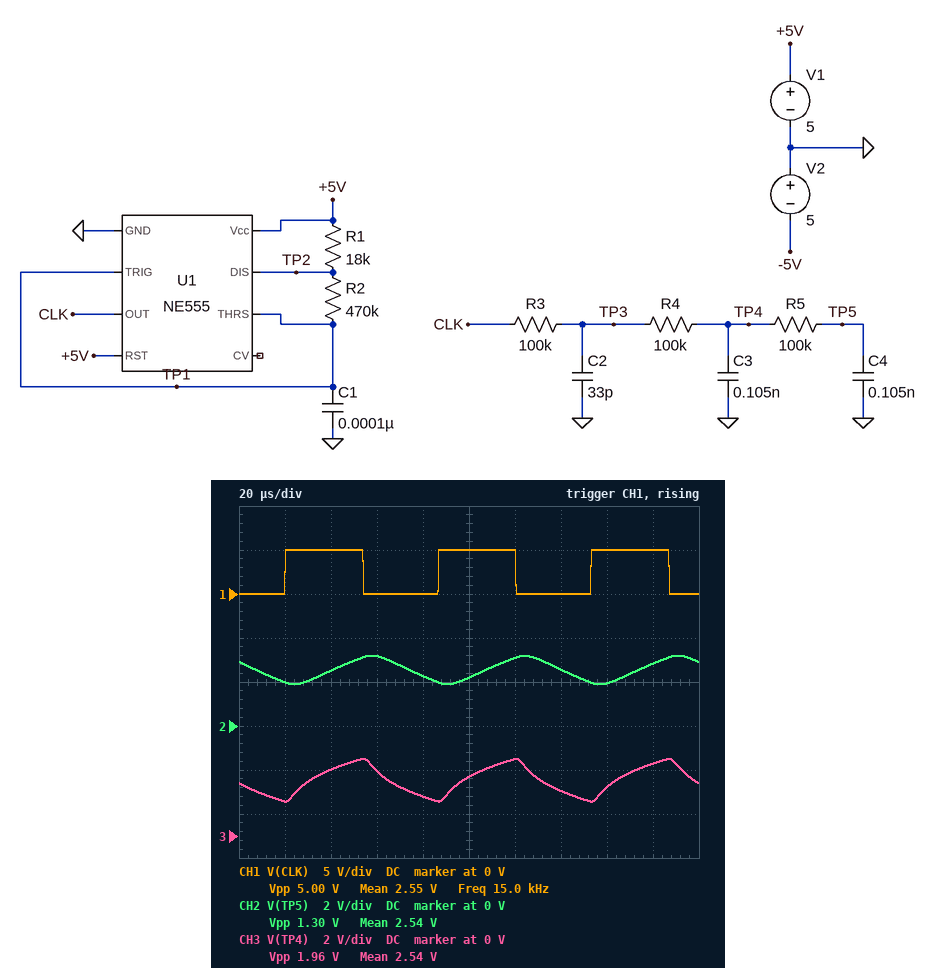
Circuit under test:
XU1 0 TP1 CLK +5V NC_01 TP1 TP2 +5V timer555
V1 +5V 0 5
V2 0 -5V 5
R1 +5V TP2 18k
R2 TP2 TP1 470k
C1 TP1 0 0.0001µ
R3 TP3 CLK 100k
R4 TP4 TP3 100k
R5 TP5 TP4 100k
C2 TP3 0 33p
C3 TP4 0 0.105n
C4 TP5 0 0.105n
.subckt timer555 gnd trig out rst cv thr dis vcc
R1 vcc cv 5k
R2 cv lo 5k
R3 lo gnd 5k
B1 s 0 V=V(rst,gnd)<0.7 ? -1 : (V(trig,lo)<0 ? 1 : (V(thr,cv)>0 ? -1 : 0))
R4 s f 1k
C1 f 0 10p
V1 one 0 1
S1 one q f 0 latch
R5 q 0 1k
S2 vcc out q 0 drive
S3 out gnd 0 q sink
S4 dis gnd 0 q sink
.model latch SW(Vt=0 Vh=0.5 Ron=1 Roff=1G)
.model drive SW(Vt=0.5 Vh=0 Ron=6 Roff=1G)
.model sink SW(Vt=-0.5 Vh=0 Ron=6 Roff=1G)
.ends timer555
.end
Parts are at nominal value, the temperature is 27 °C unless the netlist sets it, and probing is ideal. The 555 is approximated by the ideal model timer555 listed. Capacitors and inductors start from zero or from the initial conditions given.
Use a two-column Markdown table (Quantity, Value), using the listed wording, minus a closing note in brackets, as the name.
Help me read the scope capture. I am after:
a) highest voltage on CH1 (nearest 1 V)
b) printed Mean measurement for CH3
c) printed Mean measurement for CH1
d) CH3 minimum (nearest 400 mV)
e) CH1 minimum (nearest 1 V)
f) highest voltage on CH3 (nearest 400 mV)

| Quantity | Value |
|---|---|
| highest voltage on CH1 | 5 V |
| printed Mean measurement for CH3 | 2.54 V |
| printed Mean measurement for CH1 | 2.55 V |
| CH3 minimum | 1.6 V |
| CH1 minimum | 0 V |
| highest voltage on CH3 | 3.6 V |
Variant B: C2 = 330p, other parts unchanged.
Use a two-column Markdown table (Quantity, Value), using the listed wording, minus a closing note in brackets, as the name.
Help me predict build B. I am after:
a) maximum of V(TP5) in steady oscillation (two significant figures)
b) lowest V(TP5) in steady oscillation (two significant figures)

| Quantity | Value |
|---|---|
| maximum of V(TP5) in steady oscillation | 2.8 V |
| lowest V(TP5) in steady oscillation | 2.3 V |
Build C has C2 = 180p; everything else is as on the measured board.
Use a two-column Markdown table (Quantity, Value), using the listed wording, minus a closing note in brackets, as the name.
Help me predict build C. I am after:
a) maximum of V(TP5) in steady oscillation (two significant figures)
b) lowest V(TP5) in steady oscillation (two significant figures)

| Quantity | Value |
|---|---|
| maximum of V(TP5) in steady oscillation | 3.0 V |
| lowest V(TP5) in steady oscillation | 2.1 V |
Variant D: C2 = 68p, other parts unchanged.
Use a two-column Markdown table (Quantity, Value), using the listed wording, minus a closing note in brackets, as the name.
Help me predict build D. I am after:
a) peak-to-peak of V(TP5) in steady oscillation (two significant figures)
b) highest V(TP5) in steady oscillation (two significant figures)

| Quantity | Value |
|---|---|
| peak-to-peak of V(TP5) in steady oscillation | 1.2 V |
| highest V(TP5) in steady oscillation | 3.1 V |
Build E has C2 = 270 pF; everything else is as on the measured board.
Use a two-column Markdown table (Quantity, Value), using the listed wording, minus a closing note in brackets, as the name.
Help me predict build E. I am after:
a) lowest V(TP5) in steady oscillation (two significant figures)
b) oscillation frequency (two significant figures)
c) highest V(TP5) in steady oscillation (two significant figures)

| Quantity | Value |
|---|---|
| lowest V(TP5) in steady oscillation | 2.2 V |
| oscillation frequency | 15 kHz |
| highest V(TP5) in steady oscillation | 2.9 V |
